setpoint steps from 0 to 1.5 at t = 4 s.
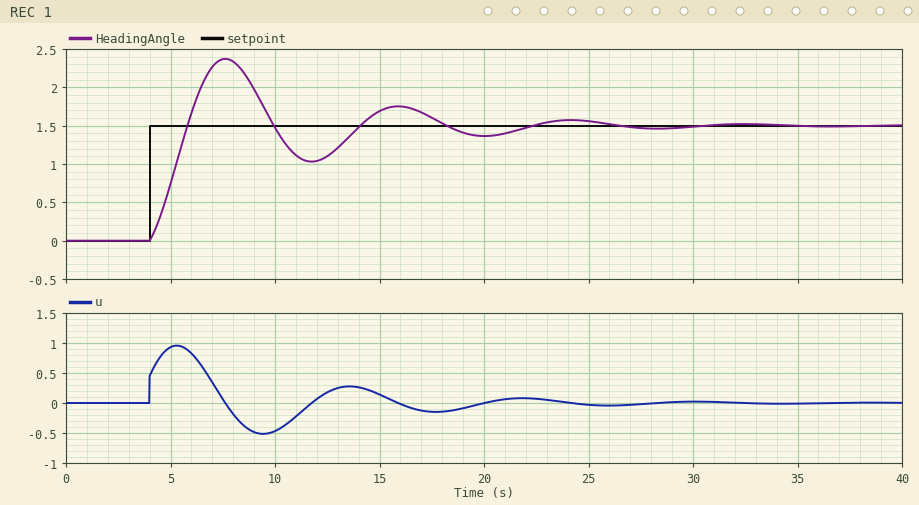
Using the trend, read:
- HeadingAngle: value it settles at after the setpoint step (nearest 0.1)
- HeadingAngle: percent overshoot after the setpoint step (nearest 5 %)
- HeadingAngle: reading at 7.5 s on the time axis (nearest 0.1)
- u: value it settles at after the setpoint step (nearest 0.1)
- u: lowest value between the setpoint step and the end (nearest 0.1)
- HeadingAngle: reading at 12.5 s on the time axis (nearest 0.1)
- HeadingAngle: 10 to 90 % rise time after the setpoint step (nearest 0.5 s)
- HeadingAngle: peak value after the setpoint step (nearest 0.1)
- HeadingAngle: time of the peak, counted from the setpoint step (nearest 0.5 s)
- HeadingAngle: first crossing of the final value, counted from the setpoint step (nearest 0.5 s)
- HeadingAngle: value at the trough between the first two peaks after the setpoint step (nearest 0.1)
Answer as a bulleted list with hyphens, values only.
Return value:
- 1.5
- 60 %
- 2.4
- 0.0
- -0.5
- 1.1
- 1.5 s
- 2.4
- 3.5 s
- 2.0 s
- 1.0
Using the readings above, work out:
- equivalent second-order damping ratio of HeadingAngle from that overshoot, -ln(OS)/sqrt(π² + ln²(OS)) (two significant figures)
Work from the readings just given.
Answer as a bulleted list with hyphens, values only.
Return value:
- 0.16
